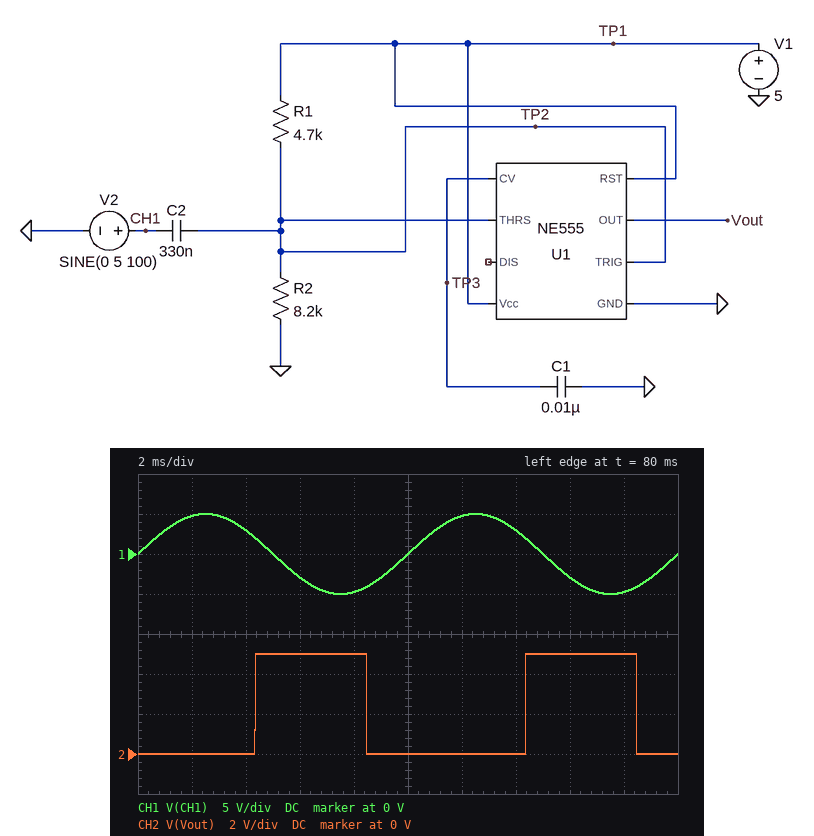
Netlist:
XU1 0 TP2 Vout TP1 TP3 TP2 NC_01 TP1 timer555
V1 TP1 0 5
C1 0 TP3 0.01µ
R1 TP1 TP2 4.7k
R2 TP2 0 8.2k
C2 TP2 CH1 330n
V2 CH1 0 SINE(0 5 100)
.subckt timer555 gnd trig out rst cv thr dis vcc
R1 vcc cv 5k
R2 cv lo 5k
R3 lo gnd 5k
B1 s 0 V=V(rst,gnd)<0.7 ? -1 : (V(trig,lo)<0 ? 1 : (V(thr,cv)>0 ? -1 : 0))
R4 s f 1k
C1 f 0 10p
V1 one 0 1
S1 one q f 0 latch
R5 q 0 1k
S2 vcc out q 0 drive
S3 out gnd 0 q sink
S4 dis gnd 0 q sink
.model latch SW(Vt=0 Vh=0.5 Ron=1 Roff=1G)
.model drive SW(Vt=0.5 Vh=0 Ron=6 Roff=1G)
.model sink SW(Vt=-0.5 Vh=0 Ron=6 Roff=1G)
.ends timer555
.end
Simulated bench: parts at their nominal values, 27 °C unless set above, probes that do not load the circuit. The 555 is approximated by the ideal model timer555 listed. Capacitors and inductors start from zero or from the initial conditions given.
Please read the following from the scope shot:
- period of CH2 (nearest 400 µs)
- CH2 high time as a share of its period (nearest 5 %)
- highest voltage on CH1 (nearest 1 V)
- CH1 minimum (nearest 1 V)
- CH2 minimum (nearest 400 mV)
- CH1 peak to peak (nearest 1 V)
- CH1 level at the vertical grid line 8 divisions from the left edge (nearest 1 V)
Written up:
10.0 ms
40 %
5 V
-5 V
0 V
10 V
-3 V
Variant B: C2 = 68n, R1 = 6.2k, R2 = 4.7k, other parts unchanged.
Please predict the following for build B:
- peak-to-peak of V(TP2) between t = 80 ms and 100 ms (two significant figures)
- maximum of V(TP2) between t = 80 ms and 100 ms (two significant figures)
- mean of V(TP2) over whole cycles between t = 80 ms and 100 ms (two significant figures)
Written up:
1.1 V
2.7 V
2.2 V
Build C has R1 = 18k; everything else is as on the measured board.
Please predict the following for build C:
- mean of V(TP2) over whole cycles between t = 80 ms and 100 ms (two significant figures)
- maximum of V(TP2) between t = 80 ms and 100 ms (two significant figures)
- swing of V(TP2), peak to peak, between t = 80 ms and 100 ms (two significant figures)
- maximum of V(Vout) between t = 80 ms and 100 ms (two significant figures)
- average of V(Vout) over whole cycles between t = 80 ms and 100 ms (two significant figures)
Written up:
1.6 V
5.4 V
7.6 V
5.0 V
2.9 V
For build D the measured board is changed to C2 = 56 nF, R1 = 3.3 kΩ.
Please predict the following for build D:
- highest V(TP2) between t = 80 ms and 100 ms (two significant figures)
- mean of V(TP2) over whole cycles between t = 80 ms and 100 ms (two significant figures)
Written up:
4.0 V
3.6 V
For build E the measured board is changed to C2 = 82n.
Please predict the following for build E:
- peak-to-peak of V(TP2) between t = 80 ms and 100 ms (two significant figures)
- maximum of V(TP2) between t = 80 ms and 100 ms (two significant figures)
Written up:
1.5 V
3.9 V
